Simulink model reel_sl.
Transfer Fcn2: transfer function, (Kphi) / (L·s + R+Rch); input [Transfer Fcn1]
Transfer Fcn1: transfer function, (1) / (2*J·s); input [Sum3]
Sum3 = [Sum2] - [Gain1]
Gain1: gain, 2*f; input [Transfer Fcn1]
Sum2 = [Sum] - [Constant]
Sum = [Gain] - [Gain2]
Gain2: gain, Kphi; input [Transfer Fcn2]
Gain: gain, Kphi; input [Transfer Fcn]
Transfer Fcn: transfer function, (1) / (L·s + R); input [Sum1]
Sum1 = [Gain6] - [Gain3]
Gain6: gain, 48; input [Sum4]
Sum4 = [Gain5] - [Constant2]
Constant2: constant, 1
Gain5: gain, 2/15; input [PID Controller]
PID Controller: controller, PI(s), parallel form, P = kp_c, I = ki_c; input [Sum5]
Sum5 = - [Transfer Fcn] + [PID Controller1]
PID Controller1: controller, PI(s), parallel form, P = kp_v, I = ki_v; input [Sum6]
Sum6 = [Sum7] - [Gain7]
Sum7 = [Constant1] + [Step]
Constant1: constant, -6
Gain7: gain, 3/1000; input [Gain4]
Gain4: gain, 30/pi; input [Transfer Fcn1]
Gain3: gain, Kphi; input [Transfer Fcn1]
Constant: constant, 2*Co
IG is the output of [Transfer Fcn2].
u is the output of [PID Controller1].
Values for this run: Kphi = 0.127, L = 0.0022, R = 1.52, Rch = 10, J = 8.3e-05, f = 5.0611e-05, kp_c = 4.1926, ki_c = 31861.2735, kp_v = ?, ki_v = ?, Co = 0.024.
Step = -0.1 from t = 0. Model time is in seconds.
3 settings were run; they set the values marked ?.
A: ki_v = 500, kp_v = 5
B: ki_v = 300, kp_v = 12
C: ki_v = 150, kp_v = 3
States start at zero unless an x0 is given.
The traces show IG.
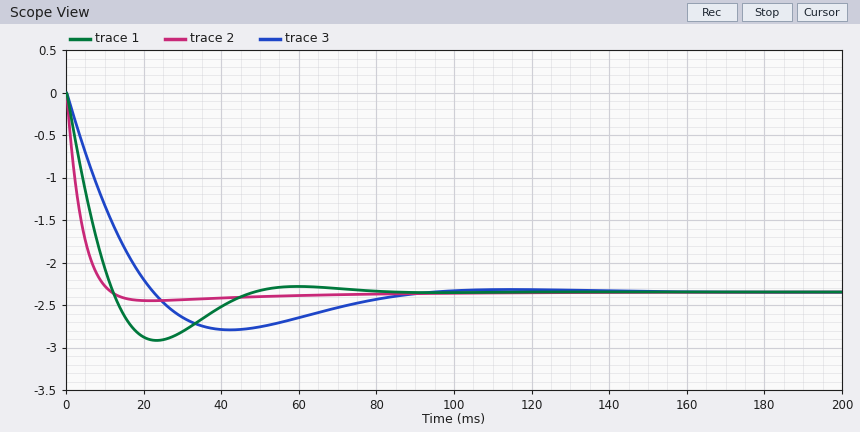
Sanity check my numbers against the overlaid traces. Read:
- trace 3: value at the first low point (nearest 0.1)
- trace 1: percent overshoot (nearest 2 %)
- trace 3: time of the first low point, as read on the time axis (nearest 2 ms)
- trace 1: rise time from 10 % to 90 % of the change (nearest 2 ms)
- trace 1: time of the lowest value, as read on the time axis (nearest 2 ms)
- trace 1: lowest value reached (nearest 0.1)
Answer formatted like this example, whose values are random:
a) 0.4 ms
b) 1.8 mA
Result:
a) -2.8
b) 24 %
c) 42 ms
d) 10 ms
e) 24 ms
f) -2.9
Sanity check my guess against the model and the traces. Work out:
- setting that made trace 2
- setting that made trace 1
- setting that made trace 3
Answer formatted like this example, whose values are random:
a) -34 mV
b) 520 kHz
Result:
a) B
b) A
c) C
